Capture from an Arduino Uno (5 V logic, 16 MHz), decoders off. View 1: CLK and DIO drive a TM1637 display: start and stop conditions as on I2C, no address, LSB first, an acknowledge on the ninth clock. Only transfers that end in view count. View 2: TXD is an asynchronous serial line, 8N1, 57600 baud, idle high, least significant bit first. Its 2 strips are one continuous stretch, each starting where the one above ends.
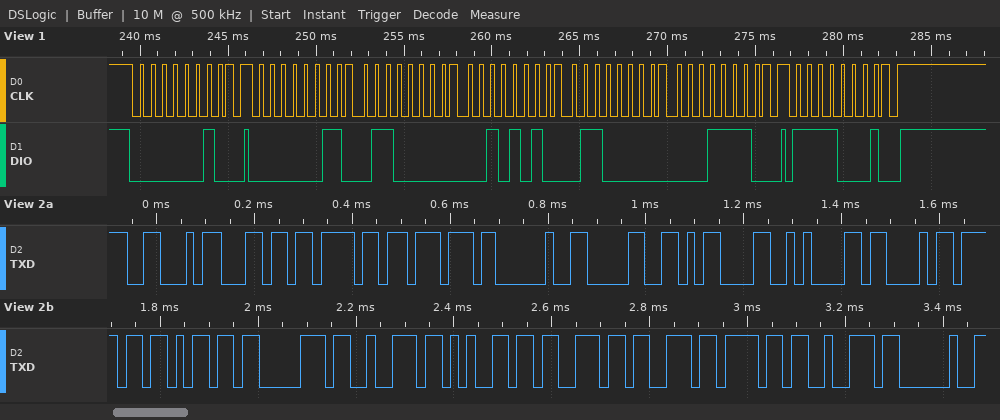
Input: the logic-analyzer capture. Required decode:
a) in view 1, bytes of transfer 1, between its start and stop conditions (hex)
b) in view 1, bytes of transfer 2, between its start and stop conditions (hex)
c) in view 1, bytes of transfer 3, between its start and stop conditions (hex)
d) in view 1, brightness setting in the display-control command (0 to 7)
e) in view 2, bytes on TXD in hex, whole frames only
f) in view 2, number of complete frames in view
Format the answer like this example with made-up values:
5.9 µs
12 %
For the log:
40
C0 06 54 06 78
8F
7
0x46 0x6C 0x6F 0x77 0x20 0x30 0x0D 0x0A 0x43 0x6F 0x6D 0x70 0x72 0x65 0x73 0x73 0x6F 0x72 0x20
19
